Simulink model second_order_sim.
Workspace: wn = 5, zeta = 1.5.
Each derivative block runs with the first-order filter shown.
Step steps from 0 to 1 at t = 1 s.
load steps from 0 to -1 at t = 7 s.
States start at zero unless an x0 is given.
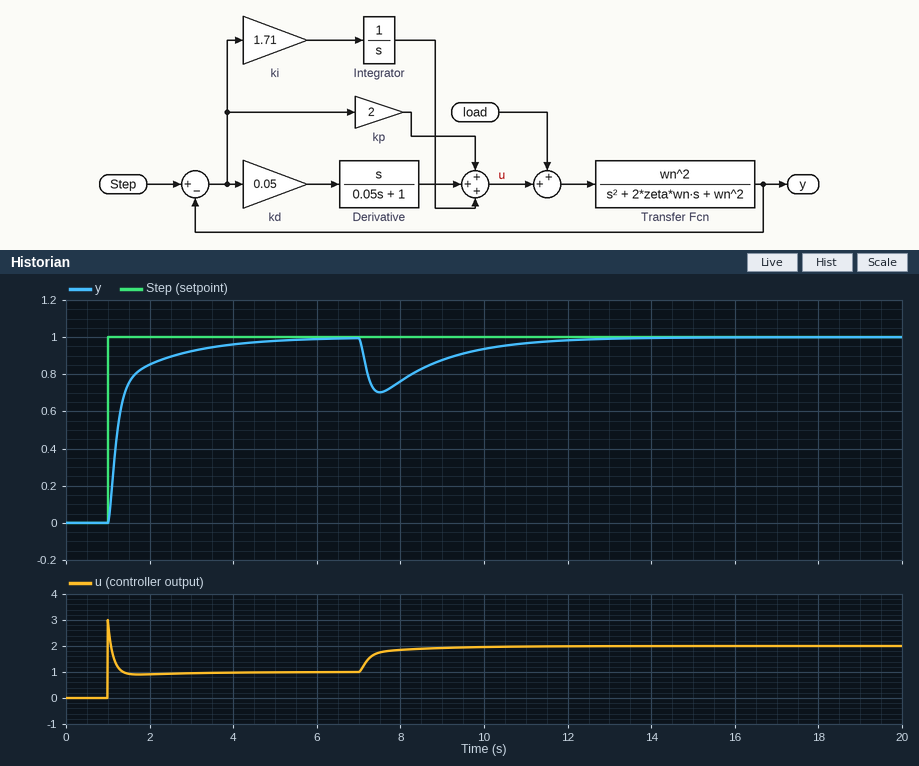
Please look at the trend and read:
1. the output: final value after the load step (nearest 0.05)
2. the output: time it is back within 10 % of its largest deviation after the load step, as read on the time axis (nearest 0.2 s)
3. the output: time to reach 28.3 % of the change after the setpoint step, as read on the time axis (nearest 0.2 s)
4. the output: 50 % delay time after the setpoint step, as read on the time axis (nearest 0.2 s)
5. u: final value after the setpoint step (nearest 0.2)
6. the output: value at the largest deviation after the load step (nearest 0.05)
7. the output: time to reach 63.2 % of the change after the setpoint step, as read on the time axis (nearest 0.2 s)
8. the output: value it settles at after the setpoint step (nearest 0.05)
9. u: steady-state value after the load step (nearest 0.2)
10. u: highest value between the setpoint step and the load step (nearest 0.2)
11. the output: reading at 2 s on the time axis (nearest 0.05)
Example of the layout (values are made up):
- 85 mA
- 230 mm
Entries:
- 1.00
- 11.2 s
- 1.2 s
- 1.2 s
- 1.0
- 0.70
- 1.4 s
- 1.00
- 2.0
- 3.0
- 0.85
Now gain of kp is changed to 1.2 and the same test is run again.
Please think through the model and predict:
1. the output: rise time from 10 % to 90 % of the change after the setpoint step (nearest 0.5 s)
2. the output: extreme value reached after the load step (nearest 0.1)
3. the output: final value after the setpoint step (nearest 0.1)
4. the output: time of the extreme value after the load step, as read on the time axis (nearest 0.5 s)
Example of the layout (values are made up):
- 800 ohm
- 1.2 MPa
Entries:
- 1.5 s
- 0.6
- 1.0
- 7.5 s
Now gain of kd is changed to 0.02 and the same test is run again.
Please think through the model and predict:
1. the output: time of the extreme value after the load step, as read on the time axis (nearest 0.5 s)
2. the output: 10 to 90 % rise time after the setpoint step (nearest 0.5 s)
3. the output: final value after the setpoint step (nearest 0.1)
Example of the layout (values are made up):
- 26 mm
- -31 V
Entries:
- 7.5 s
- 1.5 s
- 1.0
